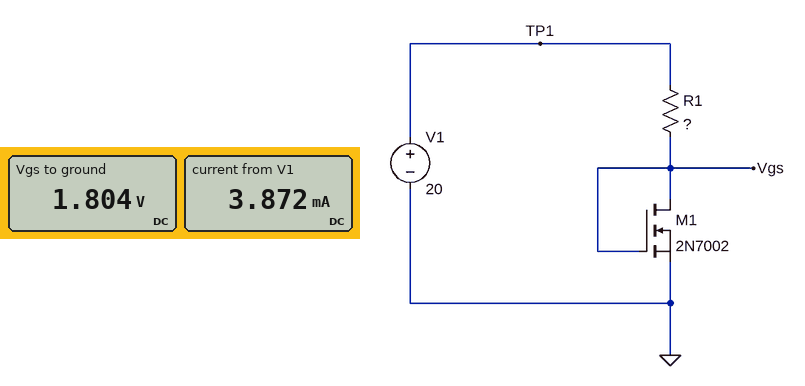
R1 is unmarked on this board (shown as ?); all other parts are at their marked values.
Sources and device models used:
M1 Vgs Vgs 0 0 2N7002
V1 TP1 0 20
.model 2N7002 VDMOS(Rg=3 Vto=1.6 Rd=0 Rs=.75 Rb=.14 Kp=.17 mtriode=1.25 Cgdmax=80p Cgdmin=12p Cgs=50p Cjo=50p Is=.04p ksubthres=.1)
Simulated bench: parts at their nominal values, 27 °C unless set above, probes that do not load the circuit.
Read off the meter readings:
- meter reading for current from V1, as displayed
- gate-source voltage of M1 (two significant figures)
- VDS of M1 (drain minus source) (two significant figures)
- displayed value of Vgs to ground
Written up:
3.872 mA
1.8 V
1.8 V
1.804 V
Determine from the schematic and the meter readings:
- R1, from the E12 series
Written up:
4.7 kΩ
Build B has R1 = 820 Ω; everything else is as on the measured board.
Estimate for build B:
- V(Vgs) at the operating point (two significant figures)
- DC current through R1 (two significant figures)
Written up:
2.1 V
22 mA
